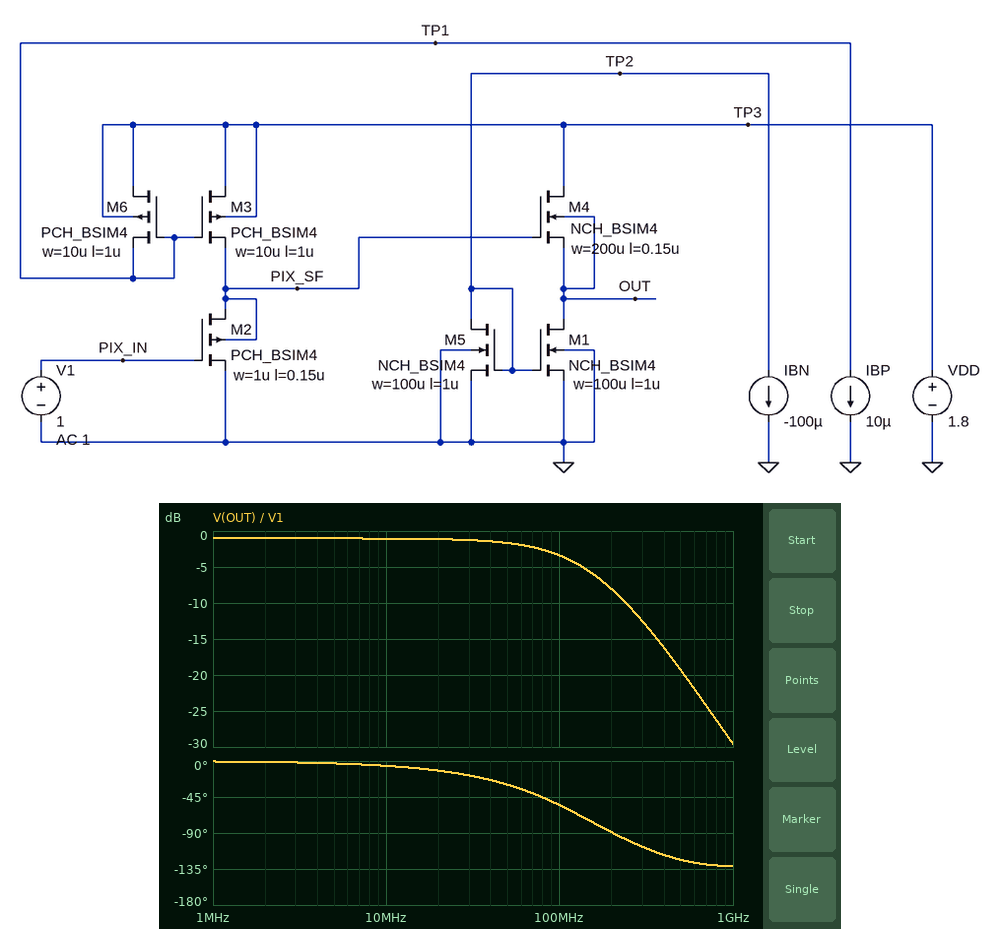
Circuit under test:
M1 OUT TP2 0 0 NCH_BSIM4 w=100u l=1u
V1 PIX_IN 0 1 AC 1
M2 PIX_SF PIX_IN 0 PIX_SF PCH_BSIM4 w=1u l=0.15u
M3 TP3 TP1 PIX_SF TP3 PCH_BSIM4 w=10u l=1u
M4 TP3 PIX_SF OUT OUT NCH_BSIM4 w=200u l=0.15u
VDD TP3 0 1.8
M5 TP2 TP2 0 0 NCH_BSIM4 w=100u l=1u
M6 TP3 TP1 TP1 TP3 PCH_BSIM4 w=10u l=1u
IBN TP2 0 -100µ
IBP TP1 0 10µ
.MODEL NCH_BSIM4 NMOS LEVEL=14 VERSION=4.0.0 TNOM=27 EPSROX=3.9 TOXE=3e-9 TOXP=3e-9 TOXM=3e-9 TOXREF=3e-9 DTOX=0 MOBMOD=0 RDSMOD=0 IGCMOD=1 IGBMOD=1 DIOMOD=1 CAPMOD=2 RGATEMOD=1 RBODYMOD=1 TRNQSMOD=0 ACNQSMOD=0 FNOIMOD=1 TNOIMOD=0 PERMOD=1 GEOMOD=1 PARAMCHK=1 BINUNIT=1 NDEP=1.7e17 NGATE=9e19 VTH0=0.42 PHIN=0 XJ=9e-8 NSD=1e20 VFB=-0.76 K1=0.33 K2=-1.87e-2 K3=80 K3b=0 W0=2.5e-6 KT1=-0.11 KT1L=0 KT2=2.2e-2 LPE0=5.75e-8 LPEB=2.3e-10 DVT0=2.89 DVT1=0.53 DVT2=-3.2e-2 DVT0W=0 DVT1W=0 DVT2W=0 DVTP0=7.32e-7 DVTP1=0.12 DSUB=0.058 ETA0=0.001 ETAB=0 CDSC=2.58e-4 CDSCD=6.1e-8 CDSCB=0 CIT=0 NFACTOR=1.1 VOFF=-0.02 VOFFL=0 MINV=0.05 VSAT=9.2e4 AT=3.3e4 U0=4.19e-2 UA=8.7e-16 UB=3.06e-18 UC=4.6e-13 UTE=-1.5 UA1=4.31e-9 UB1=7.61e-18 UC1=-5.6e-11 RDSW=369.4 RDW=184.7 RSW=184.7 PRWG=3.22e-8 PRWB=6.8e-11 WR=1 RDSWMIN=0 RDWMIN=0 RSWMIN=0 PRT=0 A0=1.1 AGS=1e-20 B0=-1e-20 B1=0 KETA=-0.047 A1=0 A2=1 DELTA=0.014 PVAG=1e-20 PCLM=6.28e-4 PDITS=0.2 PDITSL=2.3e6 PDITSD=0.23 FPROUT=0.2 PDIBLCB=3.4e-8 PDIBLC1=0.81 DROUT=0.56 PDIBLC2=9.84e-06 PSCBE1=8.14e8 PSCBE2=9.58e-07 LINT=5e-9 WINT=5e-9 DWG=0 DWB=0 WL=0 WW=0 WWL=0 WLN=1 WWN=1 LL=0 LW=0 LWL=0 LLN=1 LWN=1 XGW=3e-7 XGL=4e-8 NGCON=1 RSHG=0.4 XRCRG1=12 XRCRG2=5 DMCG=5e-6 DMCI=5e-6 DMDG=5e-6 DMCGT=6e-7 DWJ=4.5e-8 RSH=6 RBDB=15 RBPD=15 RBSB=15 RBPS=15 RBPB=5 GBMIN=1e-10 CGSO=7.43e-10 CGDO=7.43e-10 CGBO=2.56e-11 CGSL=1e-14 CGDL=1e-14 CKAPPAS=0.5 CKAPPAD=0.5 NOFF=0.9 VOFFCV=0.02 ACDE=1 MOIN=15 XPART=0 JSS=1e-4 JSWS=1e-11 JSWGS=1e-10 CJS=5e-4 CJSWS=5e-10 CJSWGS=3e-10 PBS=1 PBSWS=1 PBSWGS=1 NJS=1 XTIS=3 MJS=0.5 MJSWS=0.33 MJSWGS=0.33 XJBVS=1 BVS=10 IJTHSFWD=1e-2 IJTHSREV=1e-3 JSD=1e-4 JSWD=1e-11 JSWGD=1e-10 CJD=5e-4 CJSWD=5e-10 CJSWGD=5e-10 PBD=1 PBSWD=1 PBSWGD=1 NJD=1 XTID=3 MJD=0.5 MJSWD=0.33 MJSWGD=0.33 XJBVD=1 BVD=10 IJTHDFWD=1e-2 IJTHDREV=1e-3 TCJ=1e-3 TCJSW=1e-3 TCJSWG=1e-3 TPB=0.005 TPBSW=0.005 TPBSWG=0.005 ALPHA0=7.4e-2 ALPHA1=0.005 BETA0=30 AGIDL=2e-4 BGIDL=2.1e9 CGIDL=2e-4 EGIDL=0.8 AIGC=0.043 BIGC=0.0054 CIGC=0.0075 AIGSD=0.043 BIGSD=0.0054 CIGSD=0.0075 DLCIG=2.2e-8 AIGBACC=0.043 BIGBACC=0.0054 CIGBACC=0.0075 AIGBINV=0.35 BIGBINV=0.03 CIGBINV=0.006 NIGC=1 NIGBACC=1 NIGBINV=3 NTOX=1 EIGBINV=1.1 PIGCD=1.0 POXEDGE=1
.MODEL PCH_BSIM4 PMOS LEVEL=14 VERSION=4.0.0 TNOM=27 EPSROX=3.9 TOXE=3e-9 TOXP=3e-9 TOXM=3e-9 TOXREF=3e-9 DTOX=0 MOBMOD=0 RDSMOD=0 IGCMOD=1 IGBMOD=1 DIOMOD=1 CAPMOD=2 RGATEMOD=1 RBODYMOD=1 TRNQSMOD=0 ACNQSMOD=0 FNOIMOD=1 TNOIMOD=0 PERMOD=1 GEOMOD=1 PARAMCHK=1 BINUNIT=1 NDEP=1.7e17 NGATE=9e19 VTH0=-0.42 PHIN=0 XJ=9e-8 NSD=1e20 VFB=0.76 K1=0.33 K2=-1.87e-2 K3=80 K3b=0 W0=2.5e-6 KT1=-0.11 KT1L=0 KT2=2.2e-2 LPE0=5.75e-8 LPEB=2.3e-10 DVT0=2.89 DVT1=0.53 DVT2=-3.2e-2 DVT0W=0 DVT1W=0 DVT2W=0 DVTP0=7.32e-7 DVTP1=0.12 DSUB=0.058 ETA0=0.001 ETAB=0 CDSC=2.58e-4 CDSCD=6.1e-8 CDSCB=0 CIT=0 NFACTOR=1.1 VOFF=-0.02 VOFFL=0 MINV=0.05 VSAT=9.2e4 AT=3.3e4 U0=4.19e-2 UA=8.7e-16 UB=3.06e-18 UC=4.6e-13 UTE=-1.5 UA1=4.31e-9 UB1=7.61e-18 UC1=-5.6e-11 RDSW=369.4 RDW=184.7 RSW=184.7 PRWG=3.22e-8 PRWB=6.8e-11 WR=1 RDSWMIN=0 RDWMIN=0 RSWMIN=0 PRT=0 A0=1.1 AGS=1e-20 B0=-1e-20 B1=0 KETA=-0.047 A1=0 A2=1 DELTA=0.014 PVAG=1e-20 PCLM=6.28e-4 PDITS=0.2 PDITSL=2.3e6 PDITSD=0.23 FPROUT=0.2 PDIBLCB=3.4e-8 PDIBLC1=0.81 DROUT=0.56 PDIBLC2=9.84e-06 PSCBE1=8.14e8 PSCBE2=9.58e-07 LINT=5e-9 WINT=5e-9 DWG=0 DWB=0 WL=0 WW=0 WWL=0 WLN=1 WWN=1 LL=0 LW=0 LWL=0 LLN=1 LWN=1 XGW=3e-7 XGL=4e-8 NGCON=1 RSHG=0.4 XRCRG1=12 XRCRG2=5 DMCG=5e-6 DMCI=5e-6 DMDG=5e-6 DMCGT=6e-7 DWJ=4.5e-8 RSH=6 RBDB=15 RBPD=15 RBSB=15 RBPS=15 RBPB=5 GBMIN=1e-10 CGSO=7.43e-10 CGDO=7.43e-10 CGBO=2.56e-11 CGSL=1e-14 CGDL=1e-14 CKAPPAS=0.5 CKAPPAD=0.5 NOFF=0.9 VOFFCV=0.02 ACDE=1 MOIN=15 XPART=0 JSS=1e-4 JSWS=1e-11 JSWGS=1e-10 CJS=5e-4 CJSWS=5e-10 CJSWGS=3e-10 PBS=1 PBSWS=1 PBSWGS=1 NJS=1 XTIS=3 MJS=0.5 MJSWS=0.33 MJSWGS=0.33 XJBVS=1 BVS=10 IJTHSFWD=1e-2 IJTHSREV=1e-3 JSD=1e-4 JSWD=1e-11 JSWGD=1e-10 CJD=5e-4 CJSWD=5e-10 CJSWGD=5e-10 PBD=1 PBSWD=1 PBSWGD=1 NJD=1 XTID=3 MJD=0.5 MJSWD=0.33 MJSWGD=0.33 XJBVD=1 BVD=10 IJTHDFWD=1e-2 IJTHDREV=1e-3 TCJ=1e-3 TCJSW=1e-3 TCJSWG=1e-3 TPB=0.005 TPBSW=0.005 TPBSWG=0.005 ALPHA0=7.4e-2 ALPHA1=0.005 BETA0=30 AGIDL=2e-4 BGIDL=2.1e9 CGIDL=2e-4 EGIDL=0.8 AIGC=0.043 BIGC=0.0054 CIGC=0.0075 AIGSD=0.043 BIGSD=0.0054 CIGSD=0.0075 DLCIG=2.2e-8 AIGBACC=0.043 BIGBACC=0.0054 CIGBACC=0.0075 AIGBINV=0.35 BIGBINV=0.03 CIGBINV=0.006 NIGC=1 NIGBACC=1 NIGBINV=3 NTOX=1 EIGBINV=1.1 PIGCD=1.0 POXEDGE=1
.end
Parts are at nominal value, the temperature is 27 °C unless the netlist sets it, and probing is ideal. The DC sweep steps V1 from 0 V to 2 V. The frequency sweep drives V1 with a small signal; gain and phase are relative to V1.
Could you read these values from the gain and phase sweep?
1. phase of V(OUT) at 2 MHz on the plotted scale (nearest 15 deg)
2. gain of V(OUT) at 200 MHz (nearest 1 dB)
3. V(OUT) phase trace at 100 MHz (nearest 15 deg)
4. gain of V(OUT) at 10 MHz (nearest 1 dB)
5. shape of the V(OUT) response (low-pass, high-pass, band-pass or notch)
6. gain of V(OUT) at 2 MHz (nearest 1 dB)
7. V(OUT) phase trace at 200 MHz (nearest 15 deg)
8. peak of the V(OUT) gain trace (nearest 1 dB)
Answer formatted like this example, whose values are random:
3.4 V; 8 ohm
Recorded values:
0 deg; -8 dB; -60 deg; -1 dB; low-pass; -1 dB; -90 deg; -1 dB
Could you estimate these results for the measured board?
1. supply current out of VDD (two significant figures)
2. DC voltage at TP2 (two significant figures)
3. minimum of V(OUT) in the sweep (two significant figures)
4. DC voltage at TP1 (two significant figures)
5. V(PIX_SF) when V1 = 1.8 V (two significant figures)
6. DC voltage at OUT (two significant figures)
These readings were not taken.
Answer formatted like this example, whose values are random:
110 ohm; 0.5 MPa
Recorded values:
120 µA; 590 mV; 220 mV; 1.2 V; 1.8 V; 1.1 V
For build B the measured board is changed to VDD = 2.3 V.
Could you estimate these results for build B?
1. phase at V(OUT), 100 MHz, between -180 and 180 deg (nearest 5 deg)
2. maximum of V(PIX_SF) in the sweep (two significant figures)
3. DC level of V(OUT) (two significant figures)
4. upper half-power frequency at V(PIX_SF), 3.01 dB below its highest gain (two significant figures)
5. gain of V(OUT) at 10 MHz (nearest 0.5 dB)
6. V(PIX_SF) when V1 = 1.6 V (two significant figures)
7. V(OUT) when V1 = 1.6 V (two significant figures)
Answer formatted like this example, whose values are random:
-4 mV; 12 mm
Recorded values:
-50 deg; 2.3 V; 1.2 V; 130 MHz; -0.5 dB; 2.2 V; 1.7 V
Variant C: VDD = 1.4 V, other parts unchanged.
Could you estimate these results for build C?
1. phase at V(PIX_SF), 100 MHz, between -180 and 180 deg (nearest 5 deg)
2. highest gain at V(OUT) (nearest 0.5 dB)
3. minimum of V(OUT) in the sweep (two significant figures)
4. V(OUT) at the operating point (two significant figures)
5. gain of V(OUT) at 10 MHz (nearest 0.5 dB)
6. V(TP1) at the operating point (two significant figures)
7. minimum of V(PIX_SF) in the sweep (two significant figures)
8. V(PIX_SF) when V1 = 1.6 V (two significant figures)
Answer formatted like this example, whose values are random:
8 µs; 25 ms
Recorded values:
20 deg; -51.5 dB; 200 mV; 880 mV; -59.0 dB; 800 mV; 690 mV; 1.4 V
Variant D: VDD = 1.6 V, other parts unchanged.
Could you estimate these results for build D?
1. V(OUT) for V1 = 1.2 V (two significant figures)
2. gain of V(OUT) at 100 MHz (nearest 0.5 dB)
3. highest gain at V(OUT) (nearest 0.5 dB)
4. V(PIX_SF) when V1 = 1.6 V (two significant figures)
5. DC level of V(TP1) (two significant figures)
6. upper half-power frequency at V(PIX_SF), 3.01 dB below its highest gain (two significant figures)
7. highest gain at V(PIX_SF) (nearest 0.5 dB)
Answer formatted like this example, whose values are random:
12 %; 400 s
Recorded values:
1.1 V; -15.0 dB; -12.0 dB; 1.6 V; 1.0 V; 110 MHz; -11.5 dB
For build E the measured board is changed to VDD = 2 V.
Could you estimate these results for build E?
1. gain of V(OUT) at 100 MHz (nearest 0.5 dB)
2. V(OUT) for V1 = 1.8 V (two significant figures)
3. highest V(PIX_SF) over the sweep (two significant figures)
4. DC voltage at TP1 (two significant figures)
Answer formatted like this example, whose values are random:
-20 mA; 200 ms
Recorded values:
-3.0 dB; 1.5 V; 2.0 V; 1.4 V
